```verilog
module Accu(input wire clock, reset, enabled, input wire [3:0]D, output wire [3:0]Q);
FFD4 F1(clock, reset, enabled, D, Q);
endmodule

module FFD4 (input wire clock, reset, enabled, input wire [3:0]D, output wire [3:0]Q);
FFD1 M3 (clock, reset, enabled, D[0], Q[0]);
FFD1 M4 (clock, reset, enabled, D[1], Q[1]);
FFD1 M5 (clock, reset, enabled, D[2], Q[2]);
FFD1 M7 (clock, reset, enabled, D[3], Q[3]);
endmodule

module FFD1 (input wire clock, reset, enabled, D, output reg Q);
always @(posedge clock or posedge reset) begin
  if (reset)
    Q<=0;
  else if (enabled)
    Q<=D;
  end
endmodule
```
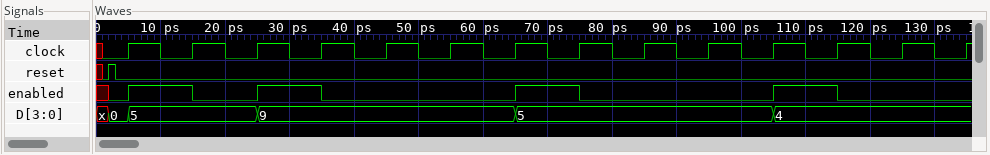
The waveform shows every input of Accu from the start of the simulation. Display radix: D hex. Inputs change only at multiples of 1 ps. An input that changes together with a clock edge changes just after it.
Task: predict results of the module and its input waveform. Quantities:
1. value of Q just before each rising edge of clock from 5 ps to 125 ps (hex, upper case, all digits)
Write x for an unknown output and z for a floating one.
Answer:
0, 0, 5, 5, 9, 9, 9, 9, 5, 5, 5, 5, 4
